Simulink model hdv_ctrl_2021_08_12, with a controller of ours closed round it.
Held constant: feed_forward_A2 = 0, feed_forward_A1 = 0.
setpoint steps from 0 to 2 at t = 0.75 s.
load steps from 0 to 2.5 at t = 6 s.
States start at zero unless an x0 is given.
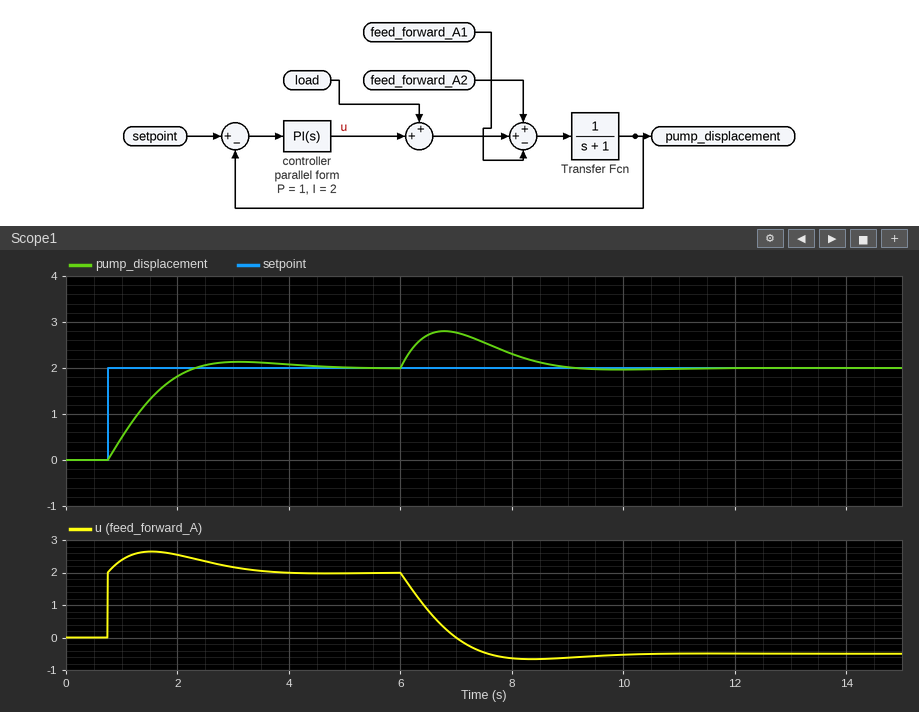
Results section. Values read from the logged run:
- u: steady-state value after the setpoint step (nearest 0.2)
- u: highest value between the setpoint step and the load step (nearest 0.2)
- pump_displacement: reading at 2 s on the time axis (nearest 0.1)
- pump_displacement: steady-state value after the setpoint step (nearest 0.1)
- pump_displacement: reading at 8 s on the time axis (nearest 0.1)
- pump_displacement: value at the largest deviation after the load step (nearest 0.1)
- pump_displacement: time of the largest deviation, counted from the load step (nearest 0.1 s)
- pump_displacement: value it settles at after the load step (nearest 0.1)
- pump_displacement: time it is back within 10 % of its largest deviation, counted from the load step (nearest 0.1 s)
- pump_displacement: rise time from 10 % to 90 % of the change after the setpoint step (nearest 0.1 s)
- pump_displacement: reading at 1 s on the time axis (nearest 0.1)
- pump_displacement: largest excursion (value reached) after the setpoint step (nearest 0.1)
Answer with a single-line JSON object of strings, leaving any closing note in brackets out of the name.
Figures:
{"u: steady-state value after the setpoint step": "2.0", "u: highest value between the setpoint step and the load step": "2.6", "pump_displacement: reading at 2 s on the time axis": "1.8", "pump_displacement: steady-state value after the setpoint step": "2.0", "pump_displacement: reading at 8 s on the time axis": "2.3", "pump_displacement: value at the largest deviation after the load step": "2.8", "pump_displacement: time of the largest deviation, counted from the load step": "0.8 s", "pump_displacement: value it settles at after the load step": "2.0", "pump_displacement: time it is back within 10 % of its largest deviation, counted from the load step": "2.7 s", "pump_displacement: rise time from 10 % to 90 % of the change after the setpoint step": "1.1 s", "pump_displacement: reading at 1 s on the time axis": "0.5", "pump_displacement: largest excursion (value reached) after the setpoint step": "2.1"}
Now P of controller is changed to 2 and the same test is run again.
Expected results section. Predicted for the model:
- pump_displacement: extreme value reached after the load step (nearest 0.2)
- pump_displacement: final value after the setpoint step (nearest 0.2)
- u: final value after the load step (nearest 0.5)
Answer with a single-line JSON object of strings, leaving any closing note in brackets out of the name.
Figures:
{"pump_displacement: extreme value reached after the load step": "2.6", "pump_displacement: final value after the setpoint step": "2.0", "u: final value after the load step": "-0.5"}
